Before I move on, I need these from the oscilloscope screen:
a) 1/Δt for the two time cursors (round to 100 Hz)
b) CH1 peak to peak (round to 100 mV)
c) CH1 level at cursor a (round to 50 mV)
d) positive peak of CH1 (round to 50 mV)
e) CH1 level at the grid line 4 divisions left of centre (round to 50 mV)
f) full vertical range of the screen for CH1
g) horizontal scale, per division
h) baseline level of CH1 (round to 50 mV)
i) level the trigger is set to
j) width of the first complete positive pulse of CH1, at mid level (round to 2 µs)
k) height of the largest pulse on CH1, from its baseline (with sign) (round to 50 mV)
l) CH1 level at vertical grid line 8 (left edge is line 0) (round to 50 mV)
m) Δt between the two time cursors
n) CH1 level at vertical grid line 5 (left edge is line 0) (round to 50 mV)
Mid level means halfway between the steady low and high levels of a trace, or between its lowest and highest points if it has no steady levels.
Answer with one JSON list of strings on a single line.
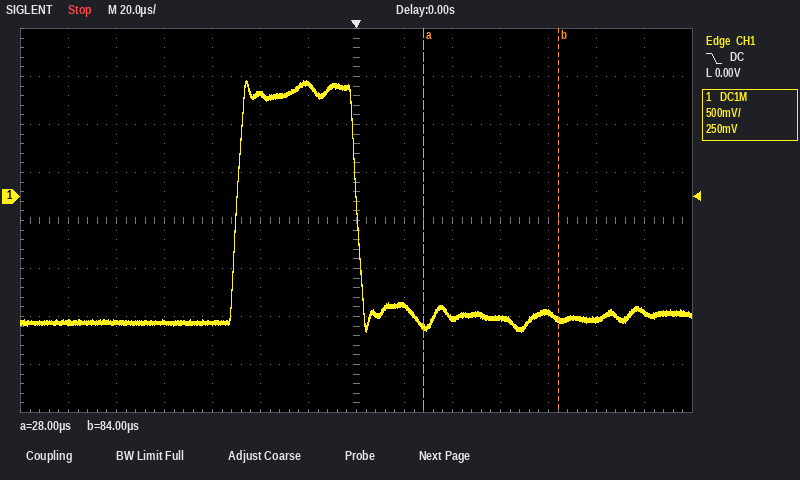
["17.9 kHz", "2.60 V", "-1.35 V", "1.20 V", "-1.30 V", "4 V", "20 µs", "-1.30 V", "0.00 V", "50 µs", "+2.50 V", "-1.15 V", "56 µs", "1.05 V"]
